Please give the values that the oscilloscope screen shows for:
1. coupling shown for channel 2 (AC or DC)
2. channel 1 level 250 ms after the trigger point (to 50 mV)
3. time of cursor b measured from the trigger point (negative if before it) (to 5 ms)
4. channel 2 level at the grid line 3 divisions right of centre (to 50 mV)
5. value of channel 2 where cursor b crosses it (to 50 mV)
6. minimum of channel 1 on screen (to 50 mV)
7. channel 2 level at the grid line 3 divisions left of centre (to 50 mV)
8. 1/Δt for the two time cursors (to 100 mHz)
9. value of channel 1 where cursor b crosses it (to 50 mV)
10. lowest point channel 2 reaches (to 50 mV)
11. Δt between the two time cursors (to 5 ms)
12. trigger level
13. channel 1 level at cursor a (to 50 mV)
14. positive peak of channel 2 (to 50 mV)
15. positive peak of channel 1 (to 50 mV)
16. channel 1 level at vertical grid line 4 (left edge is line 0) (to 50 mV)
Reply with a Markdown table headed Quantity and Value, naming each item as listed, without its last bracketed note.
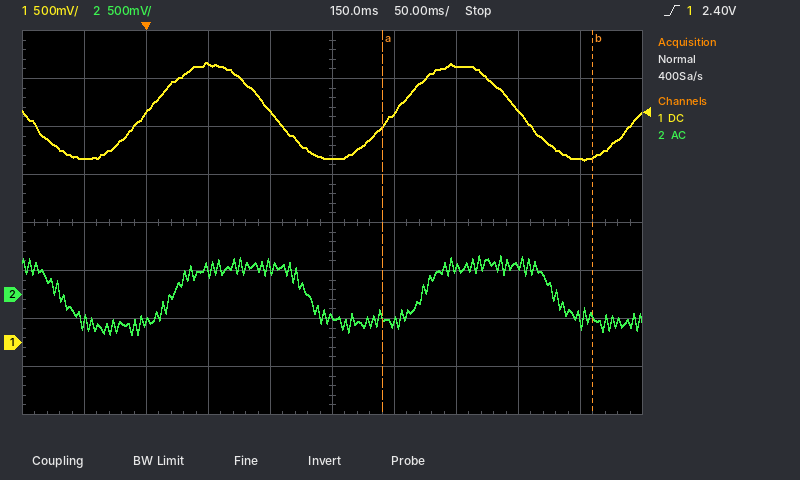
| Quantity | Value |
|---|---|
| coupling shown for channel 2 | AC |
| channel 1 level 250 ms after the trigger point | 2.90 V |
| time of cursor b measured from the trigger point (negative if before it) | +360 ms |
| channel 2 level at the grid line 3 divisions right of centre | 300 mV |
| value of channel 2 where cursor b crosses it | -250 mV |
| minimum of channel 1 on screen | 1.90 V |
| channel 2 level at the grid line 3 divisions left of centre | -300 mV |
| 1/Δt for the two time cursors | 5.9 Hz |
| value of channel 1 where cursor b crosses it | 1.95 V |
| lowest point channel 2 reaches | -400 mV |
| Δt between the two time cursors | 170 ms |
| trigger level | 2.40 V |
| channel 1 level at cursor a | 2.25 V |
| positive peak of channel 2 | 400 mV |
| positive peak of channel 1 | 2.90 V |
| channel 1 level at vertical grid line 4 (left edge is line 0) | 2.40 V |
